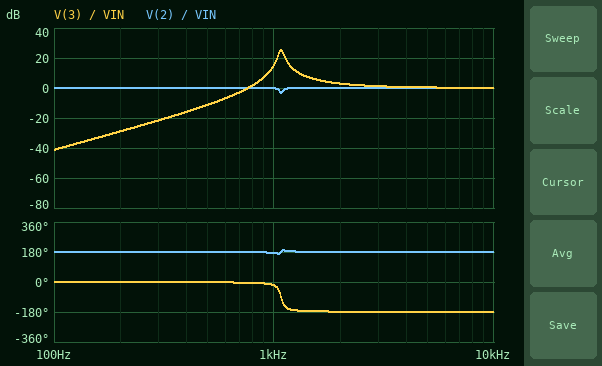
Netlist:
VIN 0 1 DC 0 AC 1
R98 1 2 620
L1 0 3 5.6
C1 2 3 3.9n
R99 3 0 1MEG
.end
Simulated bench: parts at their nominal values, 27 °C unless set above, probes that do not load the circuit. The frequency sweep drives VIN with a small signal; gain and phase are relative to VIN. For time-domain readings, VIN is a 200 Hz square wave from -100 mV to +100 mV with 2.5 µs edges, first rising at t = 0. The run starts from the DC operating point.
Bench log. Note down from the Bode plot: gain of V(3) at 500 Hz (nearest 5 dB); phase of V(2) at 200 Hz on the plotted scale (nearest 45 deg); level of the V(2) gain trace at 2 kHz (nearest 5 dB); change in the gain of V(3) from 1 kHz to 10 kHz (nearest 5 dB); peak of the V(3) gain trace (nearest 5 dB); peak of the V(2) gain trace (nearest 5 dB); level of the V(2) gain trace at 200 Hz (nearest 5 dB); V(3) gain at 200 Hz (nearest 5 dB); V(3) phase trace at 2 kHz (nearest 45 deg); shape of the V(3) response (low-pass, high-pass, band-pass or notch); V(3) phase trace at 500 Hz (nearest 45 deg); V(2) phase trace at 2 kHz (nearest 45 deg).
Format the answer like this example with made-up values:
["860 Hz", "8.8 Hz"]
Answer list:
["-10 dB", "180 deg", "0 dB", "-15 dB", "25 dB", "0 dB", "0 dB", "-30 dB", "-180 deg", "band-pass", "0 deg", "180 deg"]
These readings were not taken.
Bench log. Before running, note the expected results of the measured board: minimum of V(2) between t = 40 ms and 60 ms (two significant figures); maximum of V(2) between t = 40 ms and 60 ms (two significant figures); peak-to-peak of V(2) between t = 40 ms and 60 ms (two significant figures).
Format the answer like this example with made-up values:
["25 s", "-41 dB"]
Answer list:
["-100 mV", "100 mV", "210 mV"]
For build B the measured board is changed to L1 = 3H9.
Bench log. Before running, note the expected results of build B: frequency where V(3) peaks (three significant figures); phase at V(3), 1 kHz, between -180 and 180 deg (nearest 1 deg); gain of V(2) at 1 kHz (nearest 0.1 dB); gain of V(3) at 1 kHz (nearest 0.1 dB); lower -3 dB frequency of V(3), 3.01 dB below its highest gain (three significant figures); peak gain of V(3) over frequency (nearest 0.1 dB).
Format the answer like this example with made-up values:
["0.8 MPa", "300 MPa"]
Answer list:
["1.29 kHz", "-6 deg", "0 dB", "3.5 dB", "1.26 kHz", "25.8 dB"]
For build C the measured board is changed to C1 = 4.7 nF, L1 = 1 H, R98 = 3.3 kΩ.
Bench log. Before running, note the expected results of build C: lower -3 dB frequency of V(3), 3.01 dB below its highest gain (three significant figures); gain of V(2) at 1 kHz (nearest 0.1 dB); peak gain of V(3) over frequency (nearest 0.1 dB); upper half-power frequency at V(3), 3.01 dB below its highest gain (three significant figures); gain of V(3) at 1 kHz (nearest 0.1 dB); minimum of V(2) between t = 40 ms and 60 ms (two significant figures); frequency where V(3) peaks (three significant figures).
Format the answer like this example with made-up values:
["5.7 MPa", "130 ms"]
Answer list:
["2.11 kHz", "-0.1 dB", "12.4 dB", "2.71 kHz", "-12.9 dB", "-130 mV", "2.35 kHz"]
